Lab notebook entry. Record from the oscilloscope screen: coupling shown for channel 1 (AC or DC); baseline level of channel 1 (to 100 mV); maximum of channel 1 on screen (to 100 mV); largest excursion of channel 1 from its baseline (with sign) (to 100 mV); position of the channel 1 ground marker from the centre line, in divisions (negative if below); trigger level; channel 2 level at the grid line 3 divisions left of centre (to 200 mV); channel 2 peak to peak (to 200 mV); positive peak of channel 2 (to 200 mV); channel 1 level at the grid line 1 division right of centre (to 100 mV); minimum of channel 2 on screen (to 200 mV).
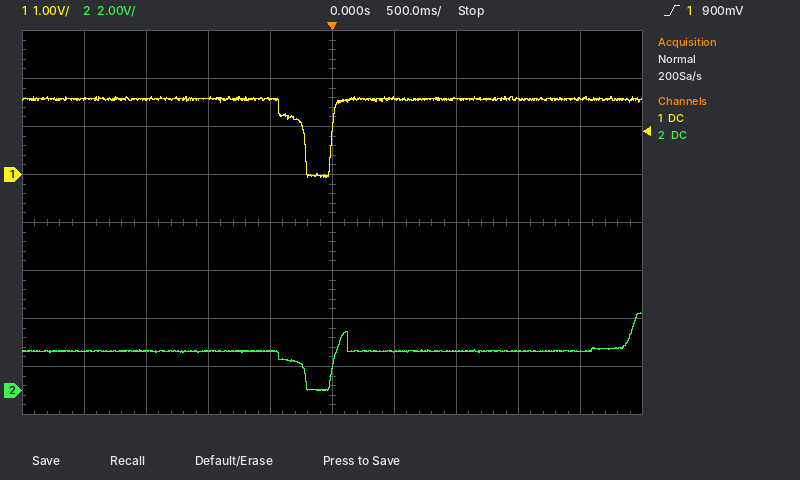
DC
1.6 V
1.6 V
-1.6 V
+1.0 div
900 mV
1.6 V
3.2 V
3.2 V
1.6 V
0.0 V
